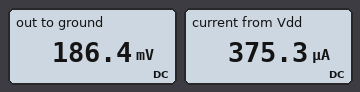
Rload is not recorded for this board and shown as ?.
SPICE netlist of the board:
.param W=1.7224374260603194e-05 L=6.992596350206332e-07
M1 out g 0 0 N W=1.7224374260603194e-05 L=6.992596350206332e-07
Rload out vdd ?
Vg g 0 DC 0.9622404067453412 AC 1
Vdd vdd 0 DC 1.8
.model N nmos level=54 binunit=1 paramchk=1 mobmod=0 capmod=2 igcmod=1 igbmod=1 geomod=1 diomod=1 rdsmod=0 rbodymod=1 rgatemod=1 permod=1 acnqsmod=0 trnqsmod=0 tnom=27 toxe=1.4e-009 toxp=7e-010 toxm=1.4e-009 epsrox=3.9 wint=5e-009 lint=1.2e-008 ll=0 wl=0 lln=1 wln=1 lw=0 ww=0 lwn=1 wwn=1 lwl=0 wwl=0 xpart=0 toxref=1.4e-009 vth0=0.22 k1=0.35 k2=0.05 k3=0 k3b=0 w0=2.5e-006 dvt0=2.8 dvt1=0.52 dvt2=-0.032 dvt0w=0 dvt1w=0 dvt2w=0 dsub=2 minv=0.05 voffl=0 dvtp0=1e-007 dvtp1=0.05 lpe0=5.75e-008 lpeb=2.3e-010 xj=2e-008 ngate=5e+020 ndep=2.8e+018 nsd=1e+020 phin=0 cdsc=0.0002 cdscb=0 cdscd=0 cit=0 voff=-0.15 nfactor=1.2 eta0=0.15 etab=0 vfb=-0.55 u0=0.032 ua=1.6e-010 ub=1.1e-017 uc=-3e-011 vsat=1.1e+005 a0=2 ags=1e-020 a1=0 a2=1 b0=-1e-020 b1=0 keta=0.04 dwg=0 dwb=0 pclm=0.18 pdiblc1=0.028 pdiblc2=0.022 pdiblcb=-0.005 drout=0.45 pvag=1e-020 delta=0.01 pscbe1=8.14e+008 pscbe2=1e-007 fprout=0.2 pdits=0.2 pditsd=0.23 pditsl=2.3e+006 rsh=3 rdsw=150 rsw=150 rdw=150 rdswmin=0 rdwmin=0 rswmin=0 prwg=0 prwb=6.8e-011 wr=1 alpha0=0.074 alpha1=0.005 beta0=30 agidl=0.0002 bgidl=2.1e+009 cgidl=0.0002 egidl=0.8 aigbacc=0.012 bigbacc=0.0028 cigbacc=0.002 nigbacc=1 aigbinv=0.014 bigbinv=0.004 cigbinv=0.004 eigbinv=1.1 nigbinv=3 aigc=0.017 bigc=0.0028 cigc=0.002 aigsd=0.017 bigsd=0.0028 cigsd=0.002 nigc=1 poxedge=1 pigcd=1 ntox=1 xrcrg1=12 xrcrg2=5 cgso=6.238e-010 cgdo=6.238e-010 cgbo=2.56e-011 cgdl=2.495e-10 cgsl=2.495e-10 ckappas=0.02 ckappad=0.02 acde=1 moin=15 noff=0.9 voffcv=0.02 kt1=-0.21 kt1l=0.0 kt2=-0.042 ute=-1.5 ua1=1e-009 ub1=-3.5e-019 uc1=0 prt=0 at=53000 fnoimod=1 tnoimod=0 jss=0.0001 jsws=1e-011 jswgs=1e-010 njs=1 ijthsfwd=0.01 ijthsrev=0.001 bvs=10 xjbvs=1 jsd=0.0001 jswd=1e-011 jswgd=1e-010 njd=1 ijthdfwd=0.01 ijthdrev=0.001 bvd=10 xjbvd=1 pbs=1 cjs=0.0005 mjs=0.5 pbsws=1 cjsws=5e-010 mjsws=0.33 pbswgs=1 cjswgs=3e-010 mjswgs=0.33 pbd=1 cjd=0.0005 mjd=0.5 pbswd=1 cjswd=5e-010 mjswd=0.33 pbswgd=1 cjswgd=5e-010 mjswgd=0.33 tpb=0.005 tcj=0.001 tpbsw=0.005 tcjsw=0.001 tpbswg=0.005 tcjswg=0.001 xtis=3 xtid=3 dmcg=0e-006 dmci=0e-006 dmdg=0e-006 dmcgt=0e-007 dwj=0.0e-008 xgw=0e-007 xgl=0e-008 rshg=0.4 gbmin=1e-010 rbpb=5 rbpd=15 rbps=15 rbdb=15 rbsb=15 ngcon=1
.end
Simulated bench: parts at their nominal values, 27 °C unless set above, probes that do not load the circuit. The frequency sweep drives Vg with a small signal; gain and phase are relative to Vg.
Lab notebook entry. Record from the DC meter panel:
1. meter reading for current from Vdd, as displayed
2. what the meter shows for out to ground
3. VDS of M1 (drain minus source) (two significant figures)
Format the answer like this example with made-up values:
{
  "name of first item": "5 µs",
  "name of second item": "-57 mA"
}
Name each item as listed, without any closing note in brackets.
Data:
{
  "meter reading for current from Vdd, as displayed": "375.3 µA",
  "what the meter shows for out to ground": "186.4 mV",
  "VDS of M1 (drain minus source)": "190 mV"
}
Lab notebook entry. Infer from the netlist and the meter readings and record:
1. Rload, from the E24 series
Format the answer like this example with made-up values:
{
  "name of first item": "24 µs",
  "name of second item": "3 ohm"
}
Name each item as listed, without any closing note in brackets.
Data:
{
  "Rload, from the E24 series": "4.3 kΩ"
}
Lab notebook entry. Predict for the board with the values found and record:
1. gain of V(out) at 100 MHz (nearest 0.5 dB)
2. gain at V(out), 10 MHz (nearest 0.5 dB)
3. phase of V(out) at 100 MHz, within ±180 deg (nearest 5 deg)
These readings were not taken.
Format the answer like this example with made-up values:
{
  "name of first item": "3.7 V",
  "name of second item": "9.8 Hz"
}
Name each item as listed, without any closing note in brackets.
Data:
{
  "gain of V(out) at 100 MHz": "-19.5 dB",
  "gain at V(out), 10 MHz": "-22.5 dB",
  "phase of V(out) at 100 MHz, within ±180 deg": "130 deg"
}
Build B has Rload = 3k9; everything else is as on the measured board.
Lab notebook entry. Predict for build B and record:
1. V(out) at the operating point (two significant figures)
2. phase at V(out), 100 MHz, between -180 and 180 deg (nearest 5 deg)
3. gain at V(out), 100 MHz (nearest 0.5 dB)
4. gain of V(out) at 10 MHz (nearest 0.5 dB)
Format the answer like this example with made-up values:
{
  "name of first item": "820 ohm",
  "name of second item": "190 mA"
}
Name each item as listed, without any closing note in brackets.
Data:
{
  "V(out) at the operating point": "210 mV",
  "phase at V(out), 100 MHz, between -180 and 180 deg": "135 deg",
  "gain at V(out), 100 MHz": "-18.0 dB",
  "gain of V(out) at 10 MHz": "-20.5 dB"
}
